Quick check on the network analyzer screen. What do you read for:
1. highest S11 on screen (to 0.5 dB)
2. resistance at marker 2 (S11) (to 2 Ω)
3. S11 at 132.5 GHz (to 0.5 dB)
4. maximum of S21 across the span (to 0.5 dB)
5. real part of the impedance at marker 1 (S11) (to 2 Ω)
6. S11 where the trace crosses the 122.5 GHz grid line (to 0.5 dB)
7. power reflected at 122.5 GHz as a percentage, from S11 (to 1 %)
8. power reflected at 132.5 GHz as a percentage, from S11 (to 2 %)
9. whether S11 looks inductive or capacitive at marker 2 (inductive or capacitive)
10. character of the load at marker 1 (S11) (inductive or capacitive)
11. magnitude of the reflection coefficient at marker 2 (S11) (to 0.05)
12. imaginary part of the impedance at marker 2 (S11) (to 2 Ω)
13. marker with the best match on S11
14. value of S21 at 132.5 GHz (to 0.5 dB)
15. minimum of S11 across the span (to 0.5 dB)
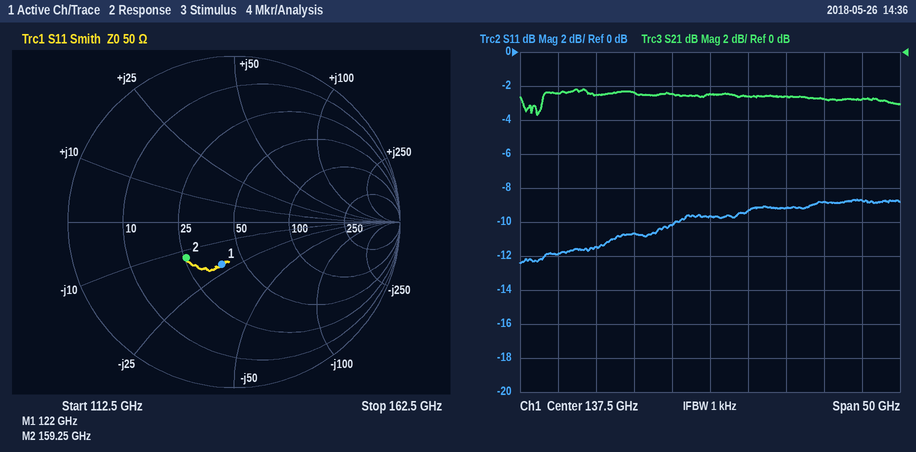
-8.5 dB
26 Ω
-10.0 dB
-2.0 dB
38 Ω
-11.5 dB
7 %
10 %
capacitive
capacitive
0.35
-12 Ω
marker 1
-2.5 dB
-12.5 dB
